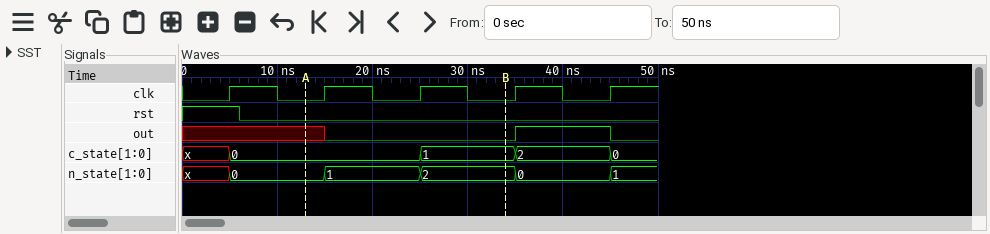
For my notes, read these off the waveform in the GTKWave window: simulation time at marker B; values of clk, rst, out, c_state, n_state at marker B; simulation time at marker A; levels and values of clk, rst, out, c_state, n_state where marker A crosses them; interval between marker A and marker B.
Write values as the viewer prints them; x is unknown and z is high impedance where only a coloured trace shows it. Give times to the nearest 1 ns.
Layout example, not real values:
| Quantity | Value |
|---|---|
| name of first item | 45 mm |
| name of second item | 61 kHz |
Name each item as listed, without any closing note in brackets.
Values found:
| Quantity | Value |
|---|---|
| simulation time at marker B | 34 ns |
| values of clk, rst, out, c_state, n_state at marker B | clk=0, rst=0, out=0, c_state=1, n_state=2 |
| simulation time at marker A | 13 ns |
| levels and values of clk, rst, out, c_state, n_state where marker A crosses them | clk=0, rst=0, out=x, c_state=0, n_state=0 |
| interval between marker A and marker B | 21 ns |
